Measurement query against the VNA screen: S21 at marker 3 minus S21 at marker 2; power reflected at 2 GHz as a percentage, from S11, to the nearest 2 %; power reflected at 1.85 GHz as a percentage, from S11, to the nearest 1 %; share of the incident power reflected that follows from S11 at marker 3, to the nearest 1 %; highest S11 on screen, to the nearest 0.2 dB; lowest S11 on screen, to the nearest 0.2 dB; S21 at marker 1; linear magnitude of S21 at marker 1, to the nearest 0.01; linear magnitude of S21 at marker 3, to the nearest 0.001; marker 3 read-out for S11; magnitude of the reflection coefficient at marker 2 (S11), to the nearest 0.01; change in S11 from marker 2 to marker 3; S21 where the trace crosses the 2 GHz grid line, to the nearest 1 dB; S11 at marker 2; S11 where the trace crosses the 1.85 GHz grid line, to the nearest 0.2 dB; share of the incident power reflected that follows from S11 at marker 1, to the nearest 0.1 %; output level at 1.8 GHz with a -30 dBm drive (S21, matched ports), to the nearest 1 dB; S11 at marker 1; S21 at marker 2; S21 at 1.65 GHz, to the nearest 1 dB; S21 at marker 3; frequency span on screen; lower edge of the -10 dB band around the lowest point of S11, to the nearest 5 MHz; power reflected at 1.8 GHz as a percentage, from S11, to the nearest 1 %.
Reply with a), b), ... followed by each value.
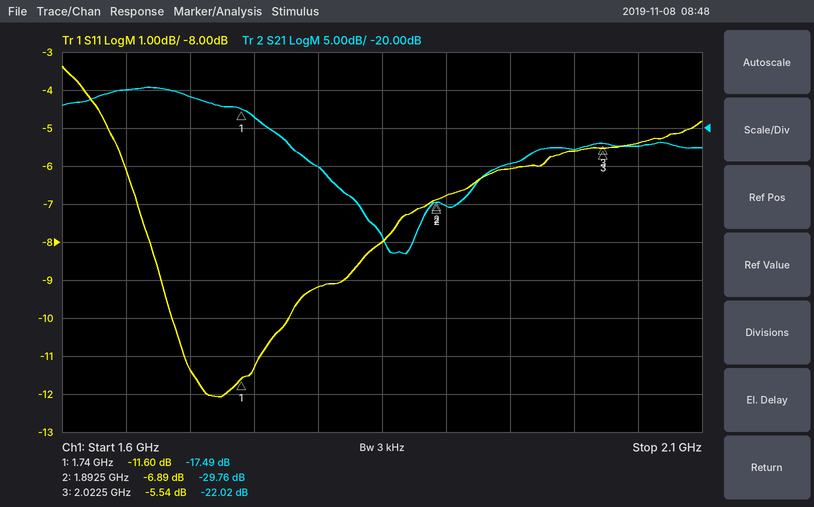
a) 7.74 dB
b) 28 %
c) 16 %
d) 28 %
e) -3.4 dB
f) -12.0 dB
g) -17.49 dB
h) 0.13
i) 0.079
j) -5.54 dB
k) 0.45
l) 1.35 dB
m) -23 dB
n) -6.89 dB
o) -8.0 dB
p) 6.9 %
q) -55 dBm
r) -11.60 dB
s) -29.76 dB
t) -15 dB
u) -22.02 dB
v) 500 MHz
w) 1.685 GHz
x) 12 %
